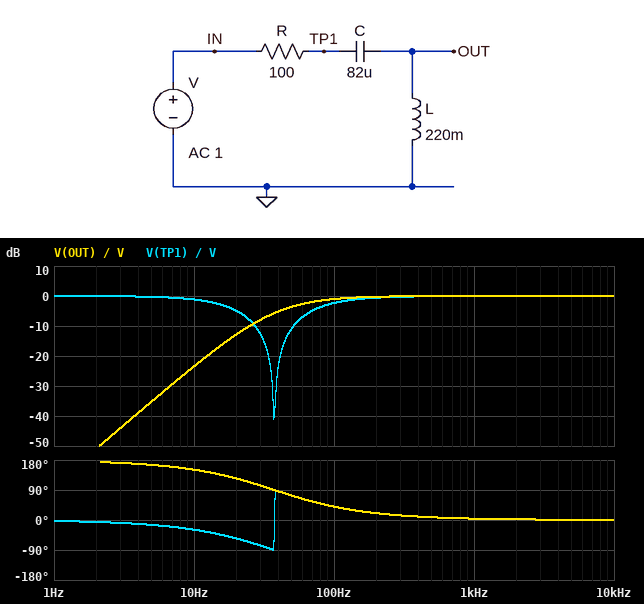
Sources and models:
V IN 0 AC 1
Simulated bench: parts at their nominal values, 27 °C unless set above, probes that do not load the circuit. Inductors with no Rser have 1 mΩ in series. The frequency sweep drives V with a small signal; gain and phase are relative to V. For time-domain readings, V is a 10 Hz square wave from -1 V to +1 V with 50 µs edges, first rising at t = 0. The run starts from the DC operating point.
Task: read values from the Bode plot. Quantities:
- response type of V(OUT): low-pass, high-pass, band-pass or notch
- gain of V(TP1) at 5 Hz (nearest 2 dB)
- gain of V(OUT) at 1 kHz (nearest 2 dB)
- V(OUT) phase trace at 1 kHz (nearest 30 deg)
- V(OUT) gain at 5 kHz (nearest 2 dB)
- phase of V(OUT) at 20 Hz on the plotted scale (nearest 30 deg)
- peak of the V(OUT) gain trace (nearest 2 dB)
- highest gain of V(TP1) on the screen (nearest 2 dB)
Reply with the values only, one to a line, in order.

high-pass
0 dB
0 dB
0 deg
0 dB
120 deg
0 dB
0 dB
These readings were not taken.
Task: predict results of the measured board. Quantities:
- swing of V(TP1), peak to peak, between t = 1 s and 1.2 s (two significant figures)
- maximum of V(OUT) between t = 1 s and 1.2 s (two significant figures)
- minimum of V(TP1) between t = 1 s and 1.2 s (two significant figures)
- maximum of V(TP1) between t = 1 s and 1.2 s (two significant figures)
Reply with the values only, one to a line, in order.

2.0 V
2.0 V
-1.0 V
1.0 V
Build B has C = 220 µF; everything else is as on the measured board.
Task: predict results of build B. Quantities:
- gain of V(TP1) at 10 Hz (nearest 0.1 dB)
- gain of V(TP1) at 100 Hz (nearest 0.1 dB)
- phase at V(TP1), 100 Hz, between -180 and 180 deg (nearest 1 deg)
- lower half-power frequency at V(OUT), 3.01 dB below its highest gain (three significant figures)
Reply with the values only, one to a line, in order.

-5.9 dB
-2.0 dB
37 deg
65.2 Hz
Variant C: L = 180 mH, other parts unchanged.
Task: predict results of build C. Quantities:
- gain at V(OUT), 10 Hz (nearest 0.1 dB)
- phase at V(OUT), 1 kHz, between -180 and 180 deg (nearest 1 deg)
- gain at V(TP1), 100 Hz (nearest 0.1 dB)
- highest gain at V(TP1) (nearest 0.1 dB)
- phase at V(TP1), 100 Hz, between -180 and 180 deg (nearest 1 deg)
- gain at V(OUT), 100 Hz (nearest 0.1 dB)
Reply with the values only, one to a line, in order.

-25.3 dB
5 deg
-3.3 dB
0 dB
47 deg
-1.7 dB
